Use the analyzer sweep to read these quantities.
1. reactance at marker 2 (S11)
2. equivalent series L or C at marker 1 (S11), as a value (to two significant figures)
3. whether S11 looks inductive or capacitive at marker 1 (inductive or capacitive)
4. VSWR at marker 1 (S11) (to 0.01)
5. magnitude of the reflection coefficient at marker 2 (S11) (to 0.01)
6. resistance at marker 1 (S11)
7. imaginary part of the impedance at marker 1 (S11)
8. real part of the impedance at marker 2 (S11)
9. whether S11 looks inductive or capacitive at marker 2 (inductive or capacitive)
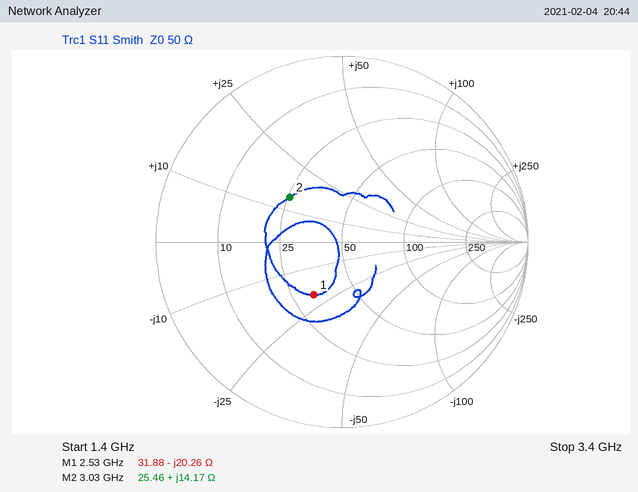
+14.17 Ω
3.1 pF
capacitive
1.95
0.37
31.88 Ω
-20.26 Ω
25.46 Ω
inductive
